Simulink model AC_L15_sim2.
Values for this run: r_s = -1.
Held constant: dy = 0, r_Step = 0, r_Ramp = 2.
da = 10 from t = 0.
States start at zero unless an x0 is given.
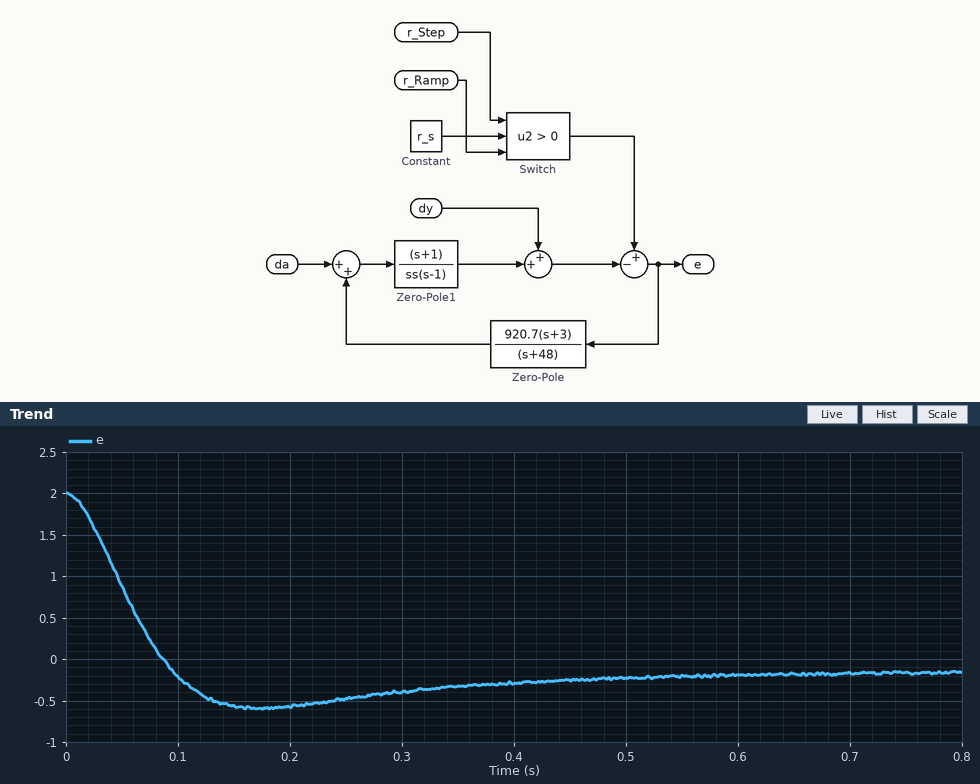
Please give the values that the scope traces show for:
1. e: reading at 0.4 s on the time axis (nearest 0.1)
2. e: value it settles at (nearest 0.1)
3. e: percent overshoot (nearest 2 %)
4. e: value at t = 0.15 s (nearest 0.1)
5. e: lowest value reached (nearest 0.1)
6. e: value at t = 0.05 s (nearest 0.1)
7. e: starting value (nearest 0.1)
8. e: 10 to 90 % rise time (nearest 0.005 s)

-0.3
-0.2
20 %
-0.6
-0.6
0.9
2.0
0.065 s
